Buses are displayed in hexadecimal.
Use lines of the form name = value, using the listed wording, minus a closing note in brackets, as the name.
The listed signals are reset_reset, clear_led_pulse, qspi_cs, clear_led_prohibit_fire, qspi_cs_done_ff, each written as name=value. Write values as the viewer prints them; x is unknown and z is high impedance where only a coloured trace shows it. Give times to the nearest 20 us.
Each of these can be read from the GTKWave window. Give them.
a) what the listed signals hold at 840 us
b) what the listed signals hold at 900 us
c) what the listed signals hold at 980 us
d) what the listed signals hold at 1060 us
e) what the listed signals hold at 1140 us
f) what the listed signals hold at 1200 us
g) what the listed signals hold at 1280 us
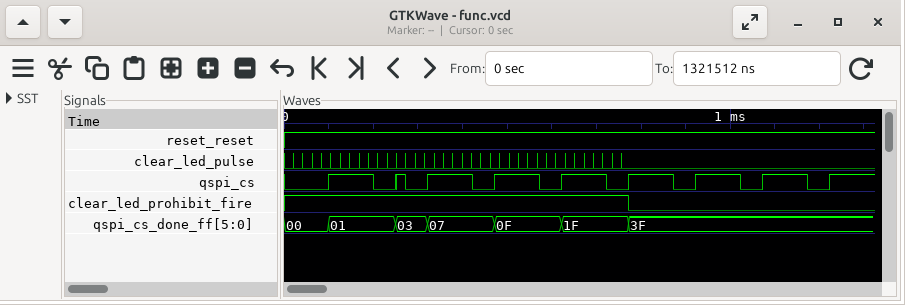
what the listed signals hold at 840 us = reset_reset=1, clear_led_pulse=0, qspi_cs=1, clear_led_prohibit_fire=0, qspi_cs_done_ff=3F
what the listed signals hold at 900 us = reset_reset=1, clear_led_pulse=0, qspi_cs=0, clear_led_prohibit_fire=0, qspi_cs_done_ff=3F
what the listed signals hold at 980 us = reset_reset=1, clear_led_pulse=0, qspi_cs=1, clear_led_prohibit_fire=0, qspi_cs_done_ff=3F
what the listed signals hold at 1060 us = reset_reset=1, clear_led_pulse=0, qspi_cs=0, clear_led_prohibit_fire=0, qspi_cs_done_ff=3F
what the listed signals hold at 1140 us = reset_reset=1, clear_led_pulse=0, qspi_cs=1, clear_led_prohibit_fire=0, qspi_cs_done_ff=3F
what the listed signals hold at 1200 us = reset_reset=1, clear_led_pulse=0, qspi_cs=0, clear_led_prohibit_fire=0, qspi_cs_done_ff=3F
what the listed signals hold at 1280 us = reset_reset=1, clear_led_pulse=0, qspi_cs=1, clear_led_prohibit_fire=0, qspi_cs_done_ff=3F
